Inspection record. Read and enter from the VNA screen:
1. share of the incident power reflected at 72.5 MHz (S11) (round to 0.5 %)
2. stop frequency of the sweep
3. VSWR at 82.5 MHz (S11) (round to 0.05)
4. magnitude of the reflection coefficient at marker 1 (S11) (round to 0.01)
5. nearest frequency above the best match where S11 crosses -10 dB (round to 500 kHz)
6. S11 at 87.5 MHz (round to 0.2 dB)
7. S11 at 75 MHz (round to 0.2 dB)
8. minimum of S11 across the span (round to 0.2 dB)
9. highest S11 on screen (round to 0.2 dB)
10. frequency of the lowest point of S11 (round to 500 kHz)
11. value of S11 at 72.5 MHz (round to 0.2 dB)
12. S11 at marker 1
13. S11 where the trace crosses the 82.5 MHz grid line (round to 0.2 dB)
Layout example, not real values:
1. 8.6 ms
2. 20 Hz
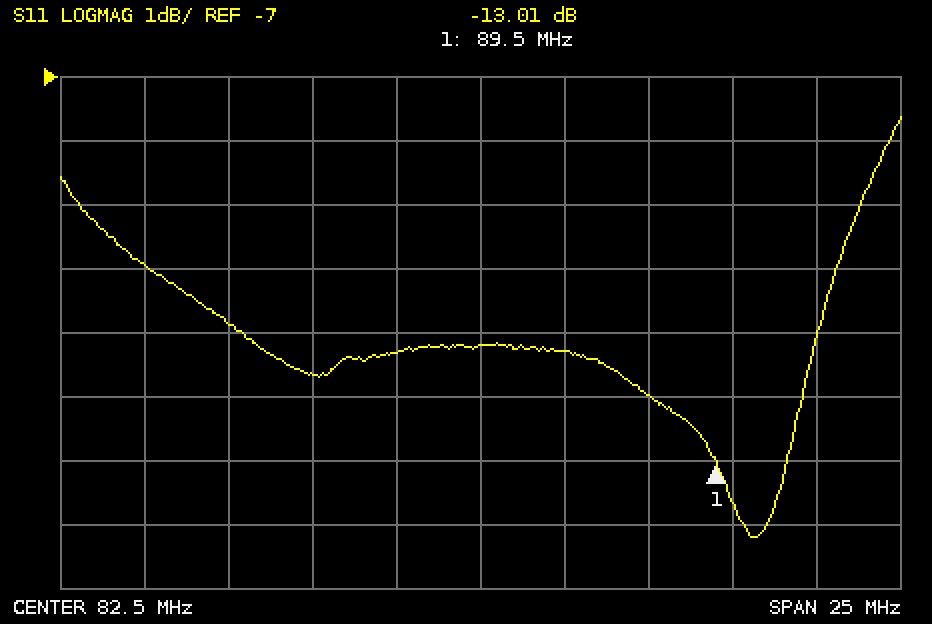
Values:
1. 10.0 %
2. 95 MHz
3. 1.75
4. 0.22
5. 93.0 MHz
6. -12.0 dB
7. -10.8 dB
8. -14.2 dB
9. -7.6 dB
10. 90.5 MHz
11. -10.0 dB
12. -13.01 dB
13. -11.2 dB
